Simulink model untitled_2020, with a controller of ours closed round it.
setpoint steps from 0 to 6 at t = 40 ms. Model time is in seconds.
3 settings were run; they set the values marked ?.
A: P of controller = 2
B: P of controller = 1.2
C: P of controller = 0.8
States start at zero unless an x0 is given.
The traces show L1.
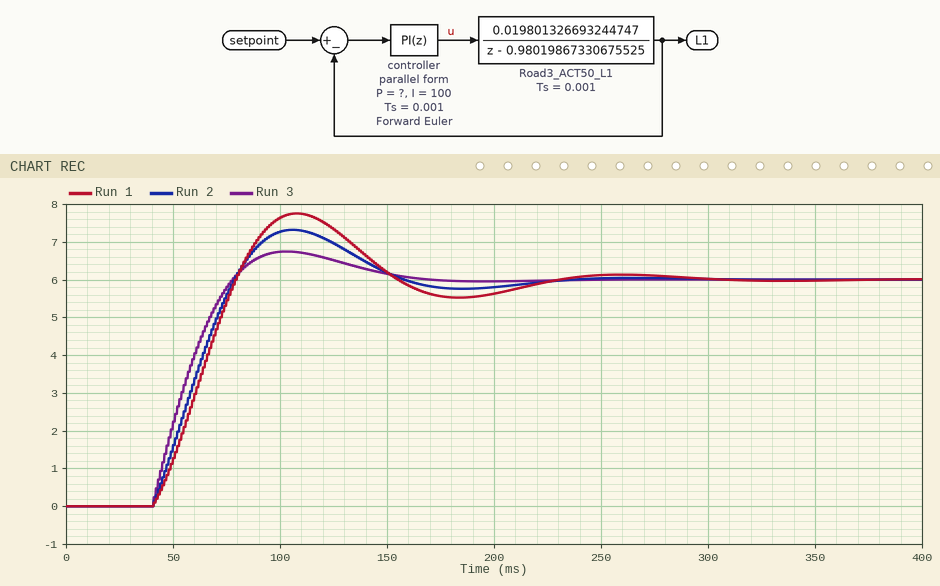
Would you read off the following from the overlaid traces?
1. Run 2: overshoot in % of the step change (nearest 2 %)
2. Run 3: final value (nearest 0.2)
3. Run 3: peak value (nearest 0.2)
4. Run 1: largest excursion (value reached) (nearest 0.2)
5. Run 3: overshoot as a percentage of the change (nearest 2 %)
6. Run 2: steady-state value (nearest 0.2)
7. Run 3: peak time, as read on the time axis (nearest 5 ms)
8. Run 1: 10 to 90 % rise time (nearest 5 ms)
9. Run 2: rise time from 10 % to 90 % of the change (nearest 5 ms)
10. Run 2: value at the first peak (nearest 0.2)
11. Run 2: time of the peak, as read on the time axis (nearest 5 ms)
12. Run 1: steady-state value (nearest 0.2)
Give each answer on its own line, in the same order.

22 %
6.0
6.8
7.8
12 %
6.0
105 ms
30 ms
30 ms
7.4
105 ms
6.0
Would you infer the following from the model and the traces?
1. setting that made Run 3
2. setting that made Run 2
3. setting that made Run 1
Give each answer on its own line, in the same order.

A
B
C
